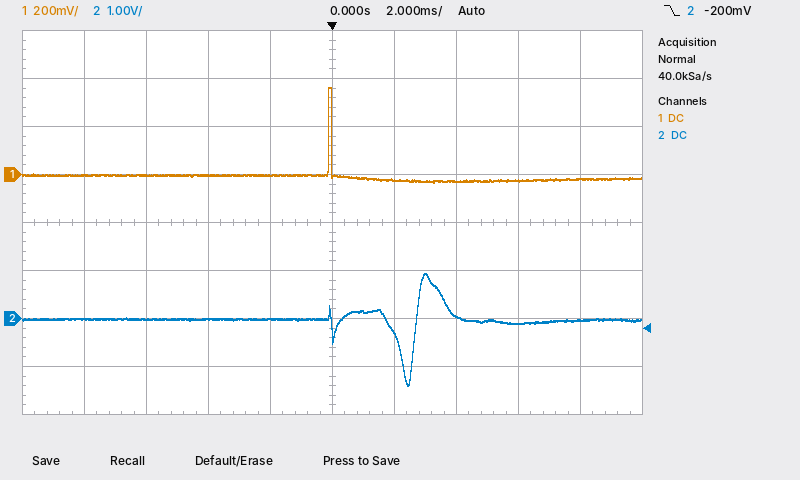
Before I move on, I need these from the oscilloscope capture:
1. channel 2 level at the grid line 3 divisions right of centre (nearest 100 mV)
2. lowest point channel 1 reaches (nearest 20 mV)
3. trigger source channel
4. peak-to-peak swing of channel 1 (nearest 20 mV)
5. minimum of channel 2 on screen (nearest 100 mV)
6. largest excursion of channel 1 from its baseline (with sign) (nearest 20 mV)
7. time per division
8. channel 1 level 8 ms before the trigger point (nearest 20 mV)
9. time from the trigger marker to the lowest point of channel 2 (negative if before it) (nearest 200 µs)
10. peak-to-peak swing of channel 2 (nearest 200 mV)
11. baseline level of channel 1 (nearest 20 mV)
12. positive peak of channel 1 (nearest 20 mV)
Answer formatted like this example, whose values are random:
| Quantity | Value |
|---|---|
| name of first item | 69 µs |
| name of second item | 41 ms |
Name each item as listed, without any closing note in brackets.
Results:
| Quantity | Value |
|---|---|
| channel 2 level at the grid line 3 divisions right of centre | -100 mV |
| lowest point channel 1 reaches | -40 mV |
| trigger source channel | channel 2 |
| peak-to-peak swing of channel 1 | 400 mV |
| minimum of channel 2 on screen | -1.4 V |
| largest excursion of channel 1 from its baseline (with sign) | +360 mV |
| time per division | 2 ms |
| channel 1 level 8 ms before the trigger point | 0 mV |
| time from the trigger marker to the lowest point of channel 2 (negative if before it) | +2.4 ms |
| peak-to-peak swing of channel 2 | 2.4 V |
| baseline level of channel 1 | 0 mV |
| positive peak of channel 1 | 360 mV |
